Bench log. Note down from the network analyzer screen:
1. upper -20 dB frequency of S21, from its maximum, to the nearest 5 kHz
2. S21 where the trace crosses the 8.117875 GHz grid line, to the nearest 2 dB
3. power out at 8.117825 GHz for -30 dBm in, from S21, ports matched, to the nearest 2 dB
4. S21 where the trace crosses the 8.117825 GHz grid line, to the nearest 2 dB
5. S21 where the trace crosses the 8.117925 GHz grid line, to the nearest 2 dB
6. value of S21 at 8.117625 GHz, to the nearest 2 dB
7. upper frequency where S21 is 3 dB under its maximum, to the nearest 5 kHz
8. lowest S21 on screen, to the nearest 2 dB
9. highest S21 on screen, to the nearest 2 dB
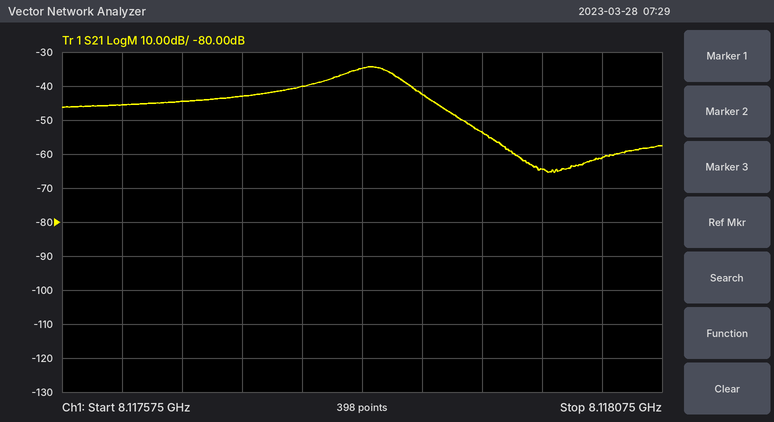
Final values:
8.117930 GHz
-42 dB
-64 dBm
-34 dB
-54 dB
-46 dB
8.117855 GHz
-66 dB
-34 dB
